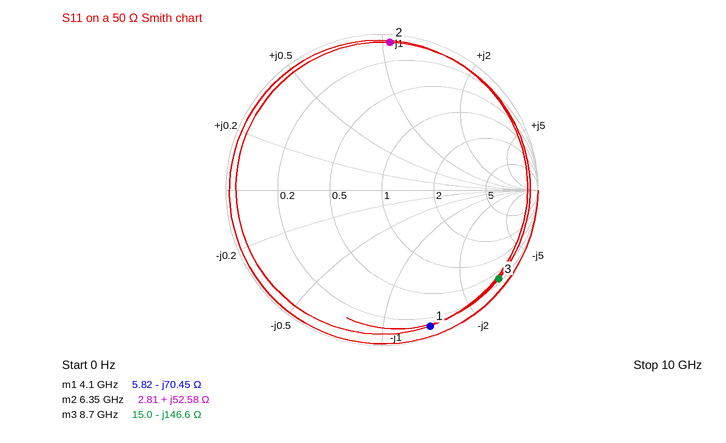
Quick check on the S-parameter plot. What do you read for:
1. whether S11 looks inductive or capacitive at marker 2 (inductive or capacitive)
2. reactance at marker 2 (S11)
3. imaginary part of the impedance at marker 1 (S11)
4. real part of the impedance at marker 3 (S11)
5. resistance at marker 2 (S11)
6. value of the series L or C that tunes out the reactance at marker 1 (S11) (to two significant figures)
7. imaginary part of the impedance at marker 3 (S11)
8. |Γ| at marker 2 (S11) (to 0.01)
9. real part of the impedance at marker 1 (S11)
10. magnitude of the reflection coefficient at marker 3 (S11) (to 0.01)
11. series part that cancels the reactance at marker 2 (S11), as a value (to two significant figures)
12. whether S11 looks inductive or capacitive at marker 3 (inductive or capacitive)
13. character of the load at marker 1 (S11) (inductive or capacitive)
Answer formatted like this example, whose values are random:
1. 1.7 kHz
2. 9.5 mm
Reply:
1. inductive
2. +52.58 Ω
3. -70.45 Ω
4. 15.0 Ω
5. 2.81 Ω
6. 2.7 nH
7. -146.6 Ω
8. 0.95
9. 5.82 Ω
10. 0.94
11. 480 fF
12. capacitive
13. capacitive
